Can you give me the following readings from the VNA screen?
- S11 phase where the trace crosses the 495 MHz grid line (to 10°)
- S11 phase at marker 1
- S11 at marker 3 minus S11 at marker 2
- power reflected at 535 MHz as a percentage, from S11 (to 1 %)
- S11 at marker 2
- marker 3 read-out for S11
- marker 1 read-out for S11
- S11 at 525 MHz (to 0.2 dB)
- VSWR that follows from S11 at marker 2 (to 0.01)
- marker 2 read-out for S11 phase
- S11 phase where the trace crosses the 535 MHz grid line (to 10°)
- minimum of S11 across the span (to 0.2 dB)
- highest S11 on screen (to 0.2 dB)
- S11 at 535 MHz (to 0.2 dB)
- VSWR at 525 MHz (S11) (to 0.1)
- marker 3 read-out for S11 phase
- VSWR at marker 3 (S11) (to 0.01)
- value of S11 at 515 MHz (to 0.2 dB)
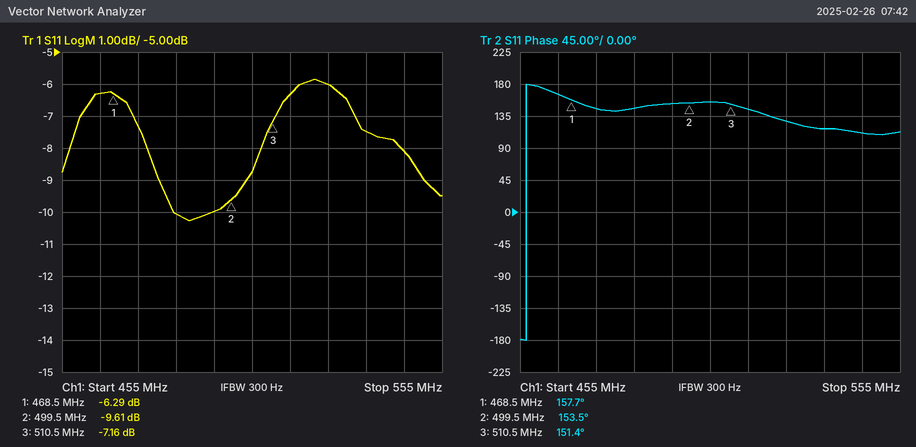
150°
157.7°
2.45 dB
18 %
-9.61 dB
-7.16 dB
-6.29 dB
-6.0 dB
1.99
153.5°
120°
-10.2 dB
-5.8 dB
-7.4 dB
3.0
151.4°
2.56
-6.4 dB
